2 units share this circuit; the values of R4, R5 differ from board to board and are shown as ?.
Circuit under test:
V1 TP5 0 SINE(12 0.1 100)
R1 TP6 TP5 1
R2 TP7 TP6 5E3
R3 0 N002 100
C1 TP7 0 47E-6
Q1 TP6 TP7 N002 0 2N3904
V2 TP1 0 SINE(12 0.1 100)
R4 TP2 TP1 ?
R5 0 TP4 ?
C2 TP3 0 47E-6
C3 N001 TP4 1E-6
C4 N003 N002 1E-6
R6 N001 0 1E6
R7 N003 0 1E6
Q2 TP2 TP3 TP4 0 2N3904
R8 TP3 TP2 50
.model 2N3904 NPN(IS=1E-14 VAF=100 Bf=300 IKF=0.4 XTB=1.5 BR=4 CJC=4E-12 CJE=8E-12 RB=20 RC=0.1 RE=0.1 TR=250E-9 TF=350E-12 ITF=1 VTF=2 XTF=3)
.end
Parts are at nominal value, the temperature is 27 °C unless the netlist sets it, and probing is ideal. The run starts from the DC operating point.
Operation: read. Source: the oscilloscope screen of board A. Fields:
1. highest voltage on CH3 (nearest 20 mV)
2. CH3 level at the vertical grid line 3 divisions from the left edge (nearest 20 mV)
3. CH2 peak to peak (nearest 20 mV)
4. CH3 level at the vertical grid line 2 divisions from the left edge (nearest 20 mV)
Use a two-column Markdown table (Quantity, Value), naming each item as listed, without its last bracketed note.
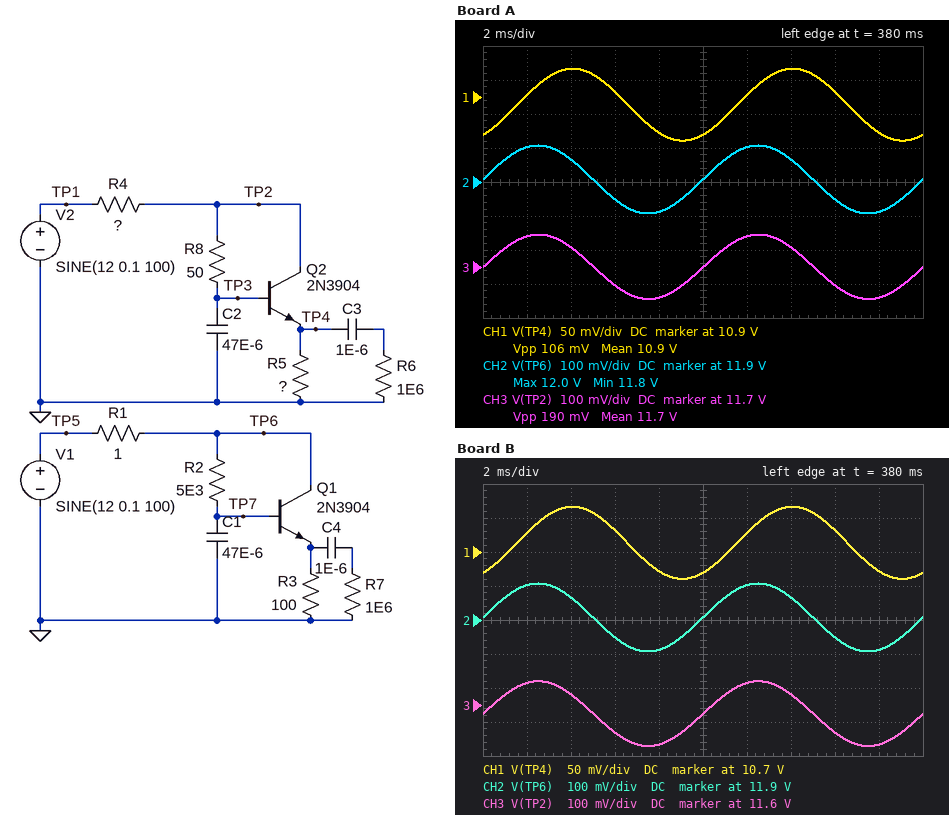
| Quantity | Value |
|---|---|
| highest voltage on CH3 | 11.80 V |
| CH3 level at the vertical grid line 3 divisions from the left edge | 11.64 V |
| CH2 peak to peak | 200 mV |
| CH3 level at the vertical grid line 2 divisions from the left edge | 11.76 V |
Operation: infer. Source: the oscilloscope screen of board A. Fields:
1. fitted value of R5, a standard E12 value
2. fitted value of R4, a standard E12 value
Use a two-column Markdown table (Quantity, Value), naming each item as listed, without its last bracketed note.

| Quantity | Value |
|---|---|
| fitted value of R5, a standard E12 value | 120 Ω |
| fitted value of R4, a standard E12 value | 3.3 Ω |
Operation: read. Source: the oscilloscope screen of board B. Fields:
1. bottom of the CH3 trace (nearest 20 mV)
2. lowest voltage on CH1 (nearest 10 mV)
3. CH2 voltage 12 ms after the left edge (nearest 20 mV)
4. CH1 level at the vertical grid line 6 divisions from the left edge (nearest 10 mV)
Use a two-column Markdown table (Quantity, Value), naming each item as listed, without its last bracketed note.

| Quantity | Value |
|---|---|
| bottom of the CH3 trace | 11.48 V |
| lowest voltage on CH1 | 10.66 V |
| CH2 voltage 12 ms after the left edge | 12.00 V |
| CH1 level at the vertical grid line 6 divisions from the left edge | 10.73 V |
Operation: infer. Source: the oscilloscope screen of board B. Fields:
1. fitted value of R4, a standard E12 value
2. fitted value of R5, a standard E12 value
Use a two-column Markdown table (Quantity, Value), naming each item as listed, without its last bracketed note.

| Quantity | Value |
|---|---|
| fitted value of R4, a standard E12 value | 2.7 Ω |
| fitted value of R5, a standard E12 value | 68 Ω |
